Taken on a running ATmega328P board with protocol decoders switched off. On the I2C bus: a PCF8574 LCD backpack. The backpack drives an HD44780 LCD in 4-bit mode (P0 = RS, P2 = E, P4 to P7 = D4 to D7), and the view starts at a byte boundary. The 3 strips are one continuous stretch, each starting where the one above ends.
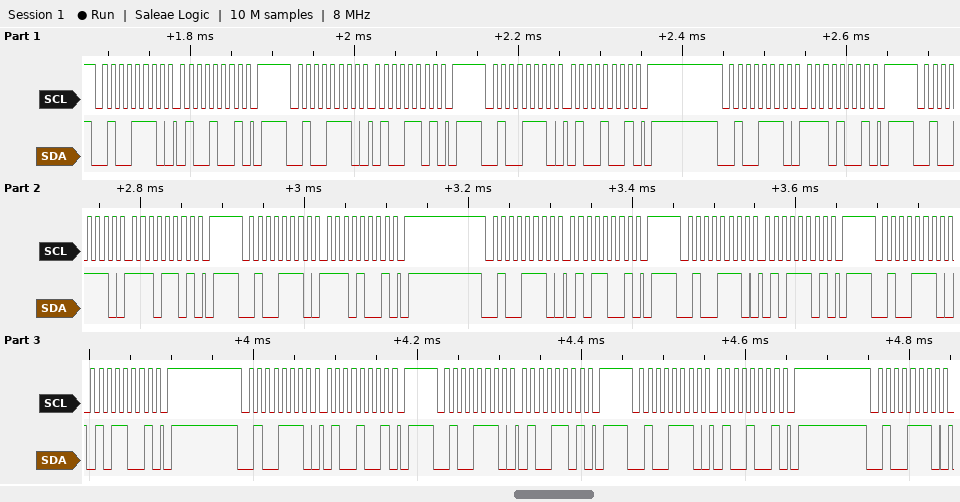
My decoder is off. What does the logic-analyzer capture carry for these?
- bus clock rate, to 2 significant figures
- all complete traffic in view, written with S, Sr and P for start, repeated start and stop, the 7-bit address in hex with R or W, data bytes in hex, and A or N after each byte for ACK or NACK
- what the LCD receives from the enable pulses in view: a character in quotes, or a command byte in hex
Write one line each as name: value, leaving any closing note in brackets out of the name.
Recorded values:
bus clock rate, to 2 significant figures: 100 kHz
all complete traffic in view, written with S, Sr and P for start, repeated start and stop, the 7-bit address in hex with R or W, data bytes in hex, and A or N after each byte for ACK or NACK: S 27W A 49 A P S 27W A 4D A P S 27W A 49 A P S 27W A E9 A P S 27W A ED A P S 27W A E9 A P S 27W A 59 A P S 27W A 5D A P S 27W A 59 A P S 27W A 49 A P S 27W A 4D A P S 27W A 49 A P S 27W A
what the LCD receives from the enable pulses in view: a character in quotes, or a command byte in hex: 'N' 'T'
